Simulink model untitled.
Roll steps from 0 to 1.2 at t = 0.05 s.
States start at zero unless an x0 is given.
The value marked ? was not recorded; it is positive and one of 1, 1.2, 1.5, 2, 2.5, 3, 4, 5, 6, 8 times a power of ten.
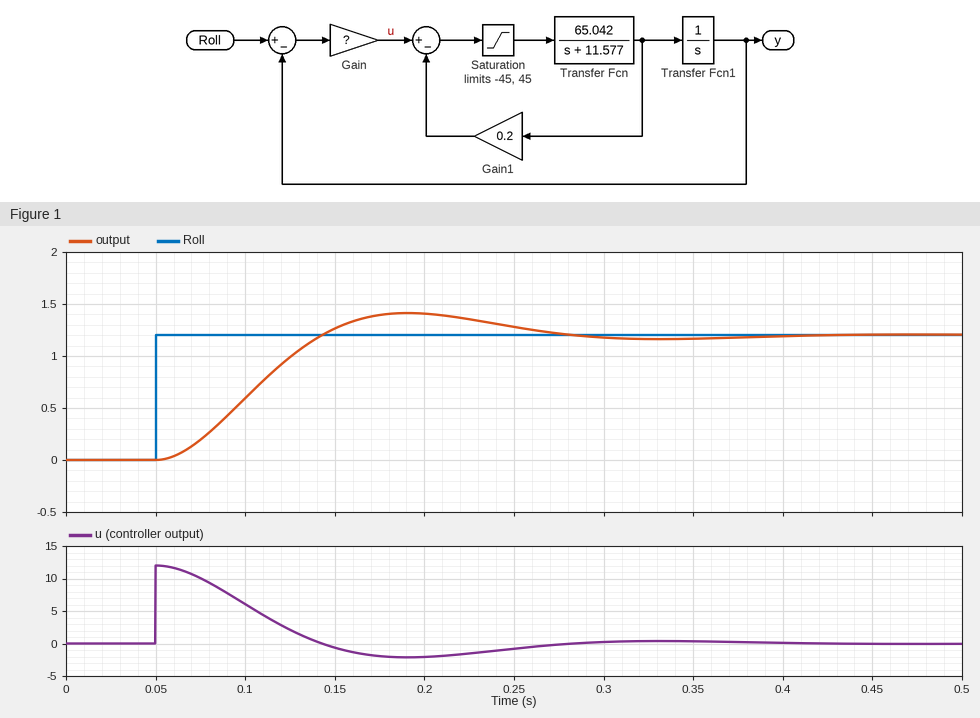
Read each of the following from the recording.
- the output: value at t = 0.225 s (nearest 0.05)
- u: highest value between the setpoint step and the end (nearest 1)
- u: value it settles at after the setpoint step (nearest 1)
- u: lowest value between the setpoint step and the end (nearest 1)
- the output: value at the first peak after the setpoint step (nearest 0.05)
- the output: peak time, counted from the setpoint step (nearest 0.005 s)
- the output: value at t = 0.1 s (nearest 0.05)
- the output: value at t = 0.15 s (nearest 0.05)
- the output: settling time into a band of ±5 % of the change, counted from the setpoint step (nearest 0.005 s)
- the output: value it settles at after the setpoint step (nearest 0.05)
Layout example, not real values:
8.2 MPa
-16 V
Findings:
1.35
12
0
-2
1.40
0.140 s
0.60
1.25
0.205 s
1.20
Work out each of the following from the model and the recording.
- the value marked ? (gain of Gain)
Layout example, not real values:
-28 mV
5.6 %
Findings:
10
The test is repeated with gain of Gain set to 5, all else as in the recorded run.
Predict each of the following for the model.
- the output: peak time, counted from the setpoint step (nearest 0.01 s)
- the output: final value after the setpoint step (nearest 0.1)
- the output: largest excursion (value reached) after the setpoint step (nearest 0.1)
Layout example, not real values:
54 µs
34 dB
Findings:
0.24 s
1.2
1.3
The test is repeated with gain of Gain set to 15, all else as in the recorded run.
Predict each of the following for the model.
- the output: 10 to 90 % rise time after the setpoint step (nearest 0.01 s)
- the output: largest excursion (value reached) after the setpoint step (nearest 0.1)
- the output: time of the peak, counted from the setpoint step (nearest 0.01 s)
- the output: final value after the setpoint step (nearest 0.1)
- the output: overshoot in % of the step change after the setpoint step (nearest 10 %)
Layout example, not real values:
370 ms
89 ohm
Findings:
0.05 s
1.5
0.11 s
1.2
30 %
